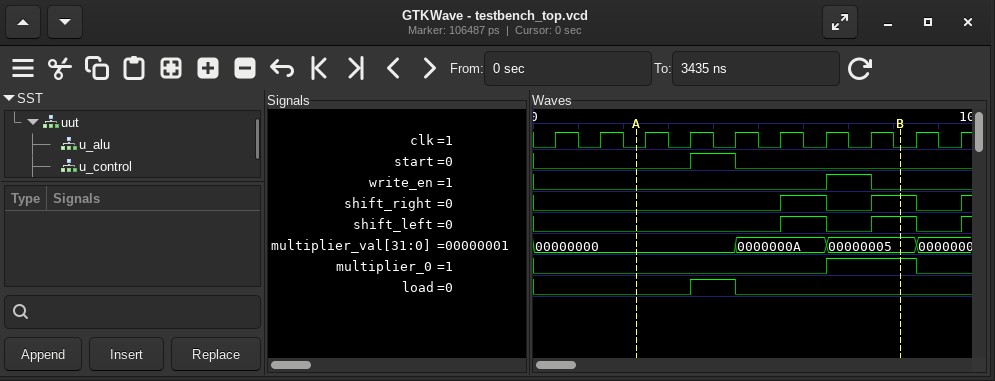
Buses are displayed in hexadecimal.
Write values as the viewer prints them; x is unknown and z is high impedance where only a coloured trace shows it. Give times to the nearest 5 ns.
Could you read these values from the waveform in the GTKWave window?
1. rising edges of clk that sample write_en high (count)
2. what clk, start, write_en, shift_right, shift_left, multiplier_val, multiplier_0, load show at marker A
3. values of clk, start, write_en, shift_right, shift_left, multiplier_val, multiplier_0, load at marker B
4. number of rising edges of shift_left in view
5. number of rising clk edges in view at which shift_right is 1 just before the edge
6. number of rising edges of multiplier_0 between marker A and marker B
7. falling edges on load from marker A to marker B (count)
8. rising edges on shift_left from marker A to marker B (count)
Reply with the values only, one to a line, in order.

1
clk=0, start=0, write_en=0, shift_right=0, shift_left=0, multiplier_val=00000000, multiplier_0=0, load=0
clk=0, start=0, write_en=0, shift_right=1, shift_left=1, multiplier_val=00000005, multiplier_0=1, load=0
3
2
1
1
2
